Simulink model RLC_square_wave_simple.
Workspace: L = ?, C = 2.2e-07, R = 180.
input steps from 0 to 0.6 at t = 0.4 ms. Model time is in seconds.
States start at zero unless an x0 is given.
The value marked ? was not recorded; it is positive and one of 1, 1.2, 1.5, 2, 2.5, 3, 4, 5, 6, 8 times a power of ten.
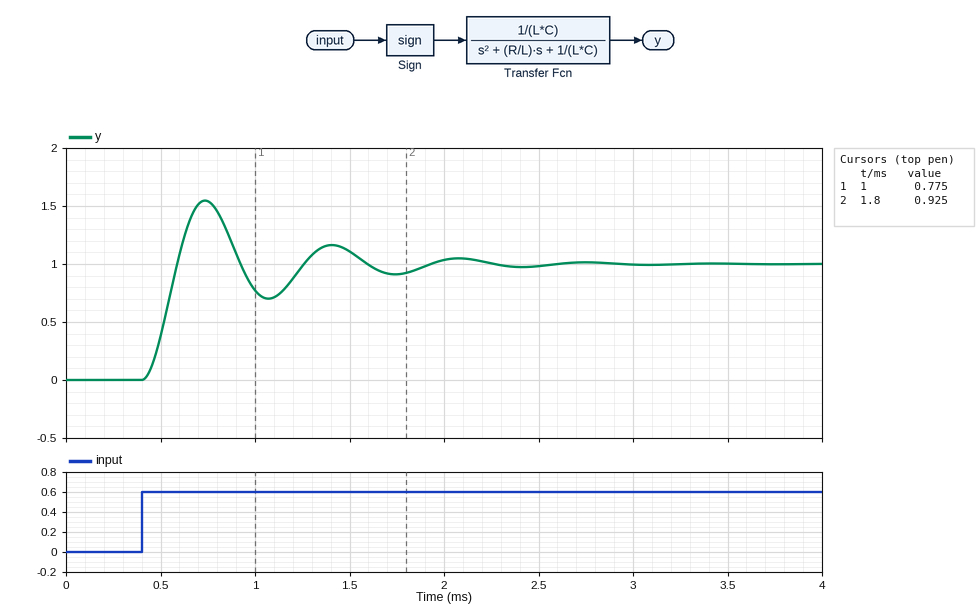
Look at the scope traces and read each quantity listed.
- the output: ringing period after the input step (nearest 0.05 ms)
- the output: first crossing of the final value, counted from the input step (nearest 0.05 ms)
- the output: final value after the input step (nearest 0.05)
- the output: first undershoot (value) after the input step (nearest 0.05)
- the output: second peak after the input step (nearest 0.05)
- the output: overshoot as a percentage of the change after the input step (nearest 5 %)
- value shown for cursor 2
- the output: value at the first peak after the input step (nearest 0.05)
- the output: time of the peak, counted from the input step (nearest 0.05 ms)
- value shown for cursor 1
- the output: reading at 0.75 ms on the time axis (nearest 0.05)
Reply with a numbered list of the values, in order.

1. 0.65 ms
2. 0.20 ms
3. 1.00
4. 0.70
5. 1.15
6. 55 %
7. 0.925
8. 1.55
9. 0.35 ms
10. 0.775
11. 1.55
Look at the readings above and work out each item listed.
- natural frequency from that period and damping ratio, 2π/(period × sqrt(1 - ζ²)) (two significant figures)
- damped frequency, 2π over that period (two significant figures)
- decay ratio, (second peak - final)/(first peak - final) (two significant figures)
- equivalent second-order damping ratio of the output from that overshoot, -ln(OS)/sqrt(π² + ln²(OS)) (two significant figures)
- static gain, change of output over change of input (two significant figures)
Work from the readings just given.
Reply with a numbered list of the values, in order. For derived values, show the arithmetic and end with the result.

1. 2π / (0.65 × sqrt(1 - 0.19²)) = 9.8 rad/ms
2. 2π / 0.65 = 9.7 rad/ms
3. (1.15 - 1) / (1.55 - 1) = 0.27
4. ln(0.55) = -0.598; 0.598 / sqrt(9.870 + 0.357) = 0.19
5. (1 - 0) / (0.6 - 0) = 1.7
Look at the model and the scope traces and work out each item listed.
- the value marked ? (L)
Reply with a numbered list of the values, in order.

1. 0.05
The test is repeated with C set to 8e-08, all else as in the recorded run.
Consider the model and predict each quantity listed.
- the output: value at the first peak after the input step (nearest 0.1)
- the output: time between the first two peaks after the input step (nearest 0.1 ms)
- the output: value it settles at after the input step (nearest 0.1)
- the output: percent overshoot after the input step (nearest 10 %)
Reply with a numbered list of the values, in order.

1. 1.7
2. 0.4 ms
3. 1.0
4. 70 %
